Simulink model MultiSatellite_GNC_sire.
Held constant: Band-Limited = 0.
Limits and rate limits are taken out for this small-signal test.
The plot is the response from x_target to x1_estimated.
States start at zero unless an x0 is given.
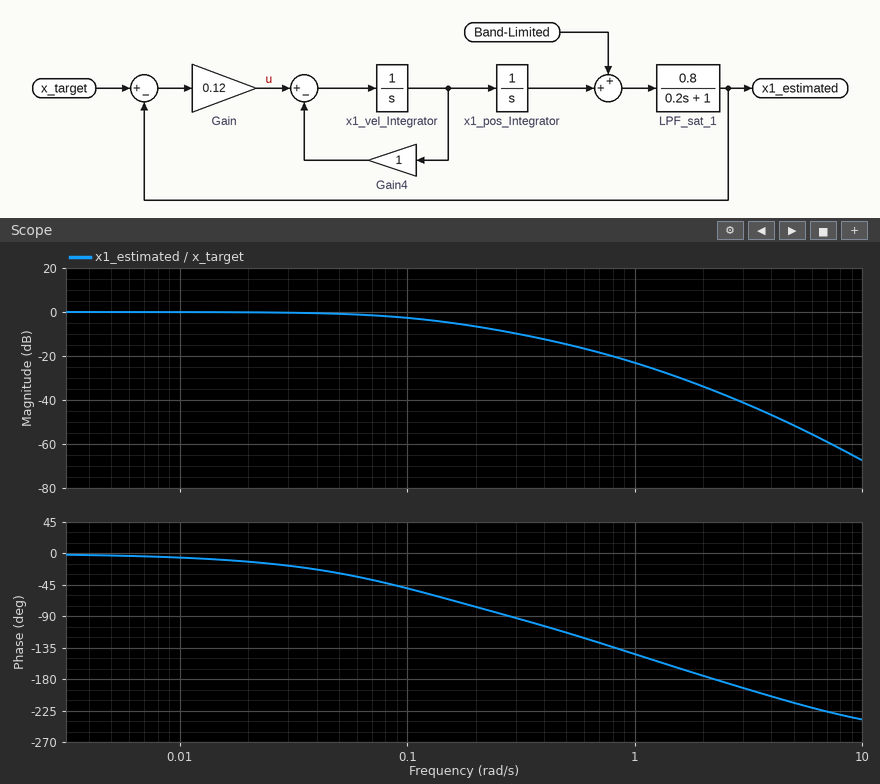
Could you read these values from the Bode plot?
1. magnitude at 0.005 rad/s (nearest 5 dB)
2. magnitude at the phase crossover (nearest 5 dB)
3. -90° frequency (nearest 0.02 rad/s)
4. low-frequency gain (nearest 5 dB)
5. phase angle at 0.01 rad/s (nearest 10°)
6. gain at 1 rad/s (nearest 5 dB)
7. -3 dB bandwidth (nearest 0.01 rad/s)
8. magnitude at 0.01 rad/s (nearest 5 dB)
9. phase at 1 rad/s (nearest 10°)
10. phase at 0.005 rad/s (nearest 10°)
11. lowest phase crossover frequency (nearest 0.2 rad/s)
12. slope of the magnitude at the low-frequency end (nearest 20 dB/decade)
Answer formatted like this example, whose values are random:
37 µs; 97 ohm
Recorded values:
0 dB; -35 dB; 0.28 rad/s; 0 dB; -10°; -25 dB; 0.11 rad/s; 0 dB; -140°; 0°; 2.2 rad/s; 0 dB/decade
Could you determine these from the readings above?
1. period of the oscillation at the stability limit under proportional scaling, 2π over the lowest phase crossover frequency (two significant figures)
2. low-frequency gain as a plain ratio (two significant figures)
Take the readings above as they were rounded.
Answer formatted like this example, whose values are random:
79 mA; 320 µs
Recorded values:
2.9 s; 1.0
